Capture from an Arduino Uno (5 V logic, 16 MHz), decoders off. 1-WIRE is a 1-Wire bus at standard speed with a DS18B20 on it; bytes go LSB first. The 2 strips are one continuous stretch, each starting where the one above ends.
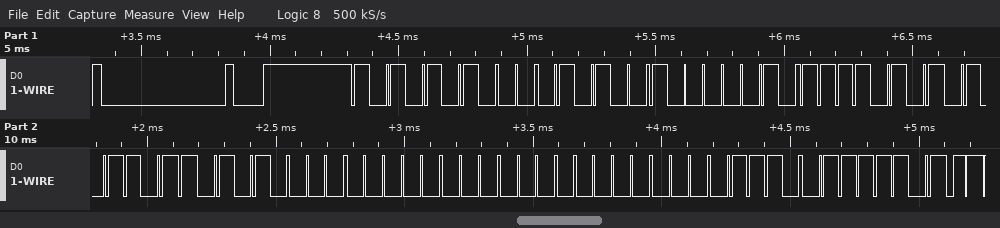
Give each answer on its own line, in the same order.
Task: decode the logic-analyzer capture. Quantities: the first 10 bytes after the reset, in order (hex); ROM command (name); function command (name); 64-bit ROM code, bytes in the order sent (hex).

55 28 41 AF DA 0A 00 00 70 BE
Match ROM
Read Scratchpad
28 41 AF DA 0A 00 00 70
